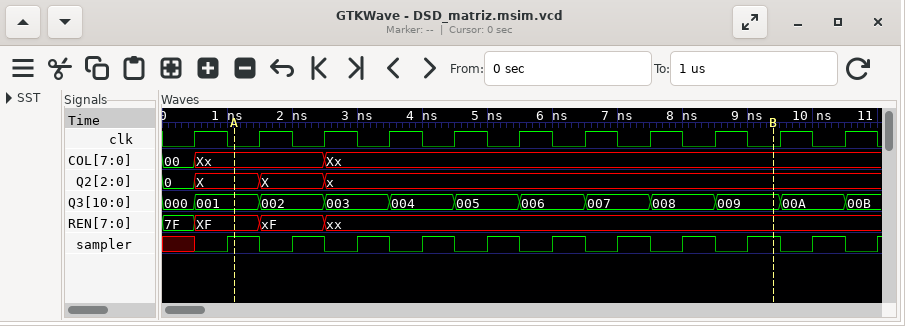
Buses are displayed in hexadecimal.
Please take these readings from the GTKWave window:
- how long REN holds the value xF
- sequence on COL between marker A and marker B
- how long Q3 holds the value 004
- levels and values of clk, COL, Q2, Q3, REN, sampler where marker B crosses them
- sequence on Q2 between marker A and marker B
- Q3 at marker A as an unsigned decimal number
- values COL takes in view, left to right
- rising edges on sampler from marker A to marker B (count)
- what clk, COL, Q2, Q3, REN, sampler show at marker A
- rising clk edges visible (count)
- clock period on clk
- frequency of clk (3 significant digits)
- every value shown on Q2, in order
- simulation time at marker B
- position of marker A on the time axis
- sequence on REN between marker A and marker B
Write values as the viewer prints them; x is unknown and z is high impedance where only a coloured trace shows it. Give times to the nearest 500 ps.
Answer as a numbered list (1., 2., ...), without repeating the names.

1. 1000 ps
2. Xx, Xx
3. 1000 ps
4. clk=0, COL=Xx, Q2=x, Q3=009, REN=xx, sampler=1
5. X, X, x
6. 1
7. 00, Xx, Xx
8. 8
9. clk=0, COL=Xx, Q2=X, Q3=001, REN=XF, sampler=1
10. 11
11. 1000 ps
12. 1.00 GHz
13. 0, X, X, x
14. 9500 ps
15. 1000 ps
16. XF, xF, xx
